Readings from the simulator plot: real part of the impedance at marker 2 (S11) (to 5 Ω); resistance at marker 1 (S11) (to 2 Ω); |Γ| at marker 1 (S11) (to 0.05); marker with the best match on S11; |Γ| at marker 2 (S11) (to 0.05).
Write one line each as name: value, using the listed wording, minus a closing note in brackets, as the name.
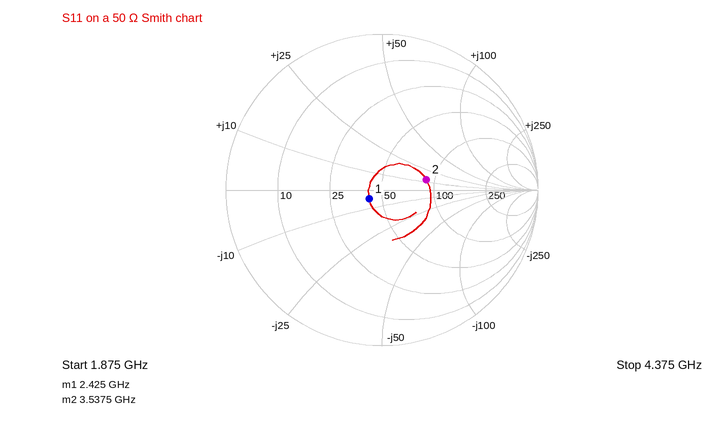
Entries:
real part of the impedance at marker 2 (S11): 90 Ω
resistance at marker 1 (S11): 42 Ω
|Γ| at marker 1 (S11): 0.10
marker with the best match on S11: marker 1
|Γ| at marker 2 (S11): 0.30
